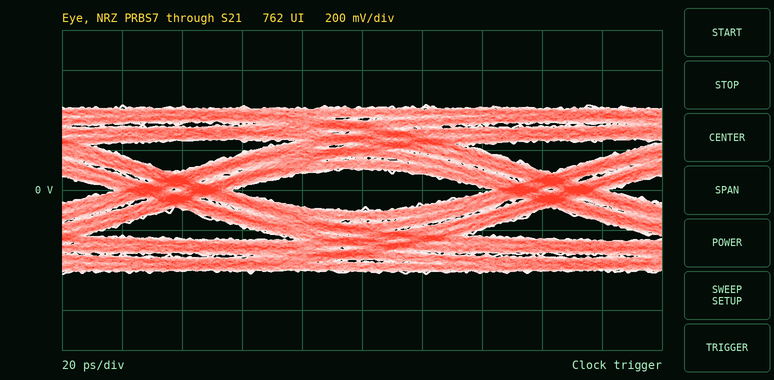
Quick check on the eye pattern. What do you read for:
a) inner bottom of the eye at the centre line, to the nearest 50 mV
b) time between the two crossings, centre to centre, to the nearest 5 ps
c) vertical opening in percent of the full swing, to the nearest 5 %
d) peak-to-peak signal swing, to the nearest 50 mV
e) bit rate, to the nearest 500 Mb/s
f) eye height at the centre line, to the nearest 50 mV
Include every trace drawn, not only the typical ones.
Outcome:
-100 mV
125 ps
25 %
850 mV
8.0 Gb/s
200 mV
